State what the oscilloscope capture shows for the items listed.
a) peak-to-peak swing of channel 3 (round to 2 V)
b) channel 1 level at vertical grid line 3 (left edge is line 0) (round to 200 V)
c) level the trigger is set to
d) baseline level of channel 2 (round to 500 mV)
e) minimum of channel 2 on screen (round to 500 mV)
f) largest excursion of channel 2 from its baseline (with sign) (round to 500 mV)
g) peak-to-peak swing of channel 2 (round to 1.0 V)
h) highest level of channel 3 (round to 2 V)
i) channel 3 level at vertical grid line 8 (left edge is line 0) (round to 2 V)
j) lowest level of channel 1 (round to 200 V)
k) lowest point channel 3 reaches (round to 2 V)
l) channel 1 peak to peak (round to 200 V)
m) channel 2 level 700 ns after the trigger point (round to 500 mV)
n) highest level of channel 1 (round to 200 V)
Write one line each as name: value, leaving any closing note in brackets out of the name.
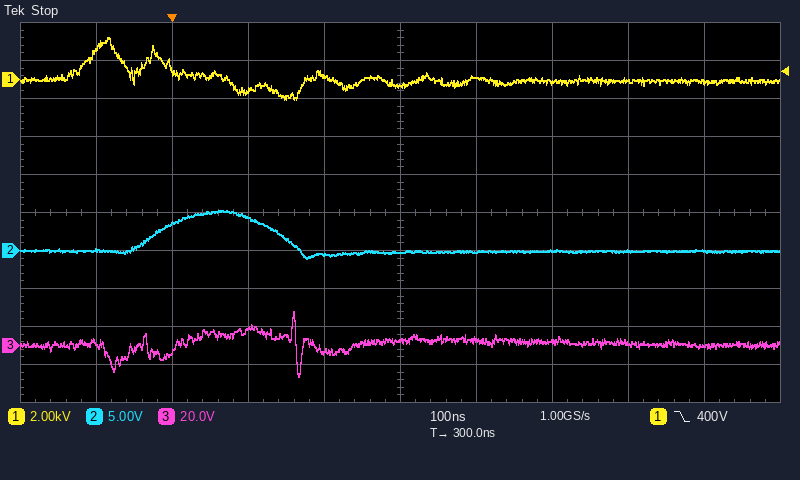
peak-to-peak swing of channel 3: 34 V
channel 1 level at vertical grid line 3 (left edge is line 0): -600 V
level the trigger is set to: 400 V
baseline level of channel 2: 0.0 V
minimum of channel 2 on screen: -1.0 V
largest excursion of channel 2 from its baseline (with sign): +5.5 V
peak-to-peak swing of channel 2: 6.0 V
highest level of channel 3: 18 V
channel 3 level at vertical grid line 8 (left edge is line 0): 2 V
lowest level of channel 1: -1.0 kV
lowest point channel 3 reaches: -16 V
channel 1 peak to peak: 3.2 kV
channel 2 level 700 ns after the trigger point: 0.0 V
highest level of channel 1: 2.2 kV
